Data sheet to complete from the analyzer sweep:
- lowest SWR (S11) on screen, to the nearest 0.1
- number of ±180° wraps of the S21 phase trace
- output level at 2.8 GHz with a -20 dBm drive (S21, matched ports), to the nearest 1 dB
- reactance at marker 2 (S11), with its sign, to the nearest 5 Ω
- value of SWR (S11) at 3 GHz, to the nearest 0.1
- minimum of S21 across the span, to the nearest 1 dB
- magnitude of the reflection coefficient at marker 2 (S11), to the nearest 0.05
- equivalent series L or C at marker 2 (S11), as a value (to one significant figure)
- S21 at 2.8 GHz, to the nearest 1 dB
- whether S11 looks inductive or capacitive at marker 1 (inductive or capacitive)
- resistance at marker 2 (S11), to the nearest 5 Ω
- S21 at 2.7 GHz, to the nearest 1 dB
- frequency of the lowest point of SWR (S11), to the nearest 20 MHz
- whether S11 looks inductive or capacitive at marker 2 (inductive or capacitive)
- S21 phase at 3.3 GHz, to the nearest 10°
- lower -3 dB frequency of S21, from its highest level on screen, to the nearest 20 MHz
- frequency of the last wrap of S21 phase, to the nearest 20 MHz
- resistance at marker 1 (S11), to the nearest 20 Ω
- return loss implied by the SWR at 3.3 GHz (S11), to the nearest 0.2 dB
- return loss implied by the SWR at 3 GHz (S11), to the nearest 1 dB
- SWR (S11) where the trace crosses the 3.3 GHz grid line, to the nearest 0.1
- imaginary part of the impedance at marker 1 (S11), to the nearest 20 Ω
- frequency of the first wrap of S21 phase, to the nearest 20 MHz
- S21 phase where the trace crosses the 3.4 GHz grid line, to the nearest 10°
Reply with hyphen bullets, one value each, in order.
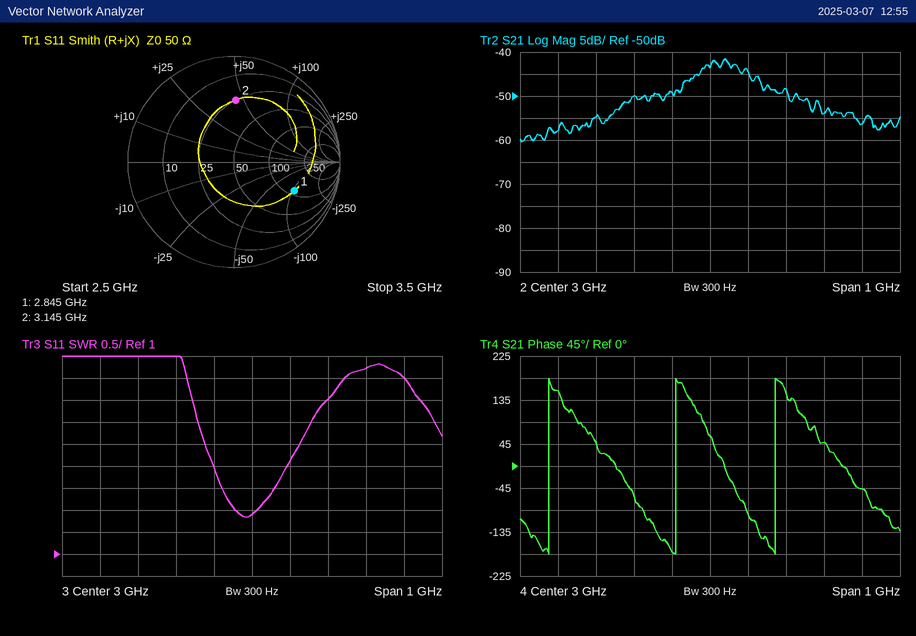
- 1.8
- 3
- -70 dBm
- +45 Ω
- 1.9
- -60 dB
- 0.60
- 2 nH
- -50 dB
- capacitive
- 25 Ω
- -55 dB
- 2.98 GHz
- inductive
- 50°
- 2.98 GHz
- 3.18 GHz
- 120 Ω
- 3.4 dB
- 10 dB
- 5.2
- -100 Ω
- 2.58 GHz
- -50°
